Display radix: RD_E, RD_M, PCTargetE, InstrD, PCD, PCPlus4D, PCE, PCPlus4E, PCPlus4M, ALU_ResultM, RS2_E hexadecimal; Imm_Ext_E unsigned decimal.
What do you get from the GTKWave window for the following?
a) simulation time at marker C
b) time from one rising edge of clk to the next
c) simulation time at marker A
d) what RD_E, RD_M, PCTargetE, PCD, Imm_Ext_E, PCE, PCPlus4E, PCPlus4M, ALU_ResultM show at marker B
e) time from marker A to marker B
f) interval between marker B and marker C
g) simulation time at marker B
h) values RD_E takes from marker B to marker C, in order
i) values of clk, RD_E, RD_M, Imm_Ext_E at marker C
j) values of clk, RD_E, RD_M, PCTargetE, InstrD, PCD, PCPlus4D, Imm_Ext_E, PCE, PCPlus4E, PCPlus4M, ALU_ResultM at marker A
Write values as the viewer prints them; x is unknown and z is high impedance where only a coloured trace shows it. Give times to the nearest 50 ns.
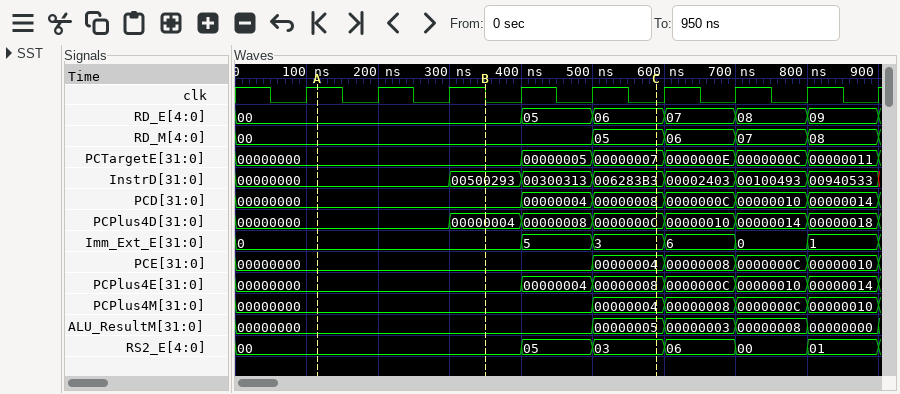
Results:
600 ns
100 ns
100 ns
RD_E=00, RD_M=00, PCTargetE=00000000, PCD=00000000, Imm_Ext_E=0, PCE=00000000, PCPlus4E=00000000, PCPlus4M=00000000, ALU_ResultM=00000000
250 ns
250 ns
350 ns
00, 05, 06
clk=0, RD_E=06, RD_M=05, Imm_Ext_E=3
clk=1, RD_E=00, RD_M=00, PCTargetE=00000000, InstrD=00000000, PCD=00000000, PCPlus4D=00000000, Imm_Ext_E=0, PCE=00000000, PCPlus4E=00000000, PCPlus4M=00000000, ALU_ResultM=00000000
